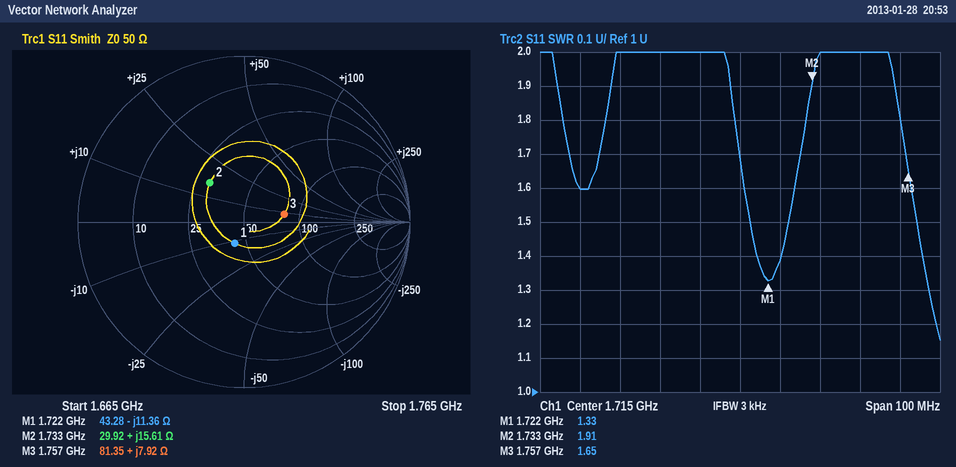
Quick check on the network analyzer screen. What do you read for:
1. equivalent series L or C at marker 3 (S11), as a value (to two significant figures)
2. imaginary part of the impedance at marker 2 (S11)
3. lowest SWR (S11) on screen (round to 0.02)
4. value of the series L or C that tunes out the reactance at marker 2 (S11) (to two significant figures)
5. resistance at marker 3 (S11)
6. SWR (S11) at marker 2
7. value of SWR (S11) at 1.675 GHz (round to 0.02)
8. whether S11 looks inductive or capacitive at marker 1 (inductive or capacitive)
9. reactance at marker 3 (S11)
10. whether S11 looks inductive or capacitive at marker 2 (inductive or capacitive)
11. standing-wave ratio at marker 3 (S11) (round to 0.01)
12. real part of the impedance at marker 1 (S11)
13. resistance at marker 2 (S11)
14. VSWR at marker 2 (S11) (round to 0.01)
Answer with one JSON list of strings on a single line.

["720 pH", "+15.61 Ω", "1.16", "5.9 pF", "81.35 Ω", "1.91", "1.60", "capacitive", "+7.92 Ω", "inductive", "1.65", "43.28 Ω", "29.92 Ω", "1.91"]
